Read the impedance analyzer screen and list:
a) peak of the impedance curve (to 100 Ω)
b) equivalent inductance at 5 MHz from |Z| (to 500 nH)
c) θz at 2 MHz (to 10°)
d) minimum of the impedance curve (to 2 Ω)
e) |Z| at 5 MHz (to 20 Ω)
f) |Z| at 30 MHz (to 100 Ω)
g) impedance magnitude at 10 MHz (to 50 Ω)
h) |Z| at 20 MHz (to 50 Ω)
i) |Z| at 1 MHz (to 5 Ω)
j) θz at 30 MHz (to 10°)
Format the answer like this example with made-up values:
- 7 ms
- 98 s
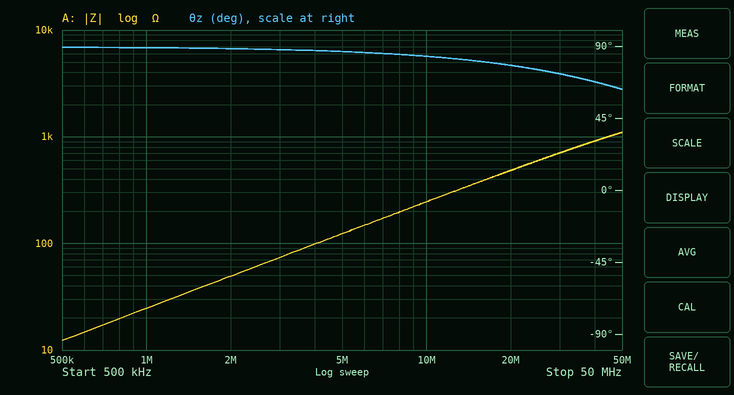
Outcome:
- 1.1 kΩ
- 4.0 µH
- 90°
- 12 Ω
- 120 Ω
- 700 Ω
- 250 Ω
- 500 Ω
- 25 Ω
- 70°
